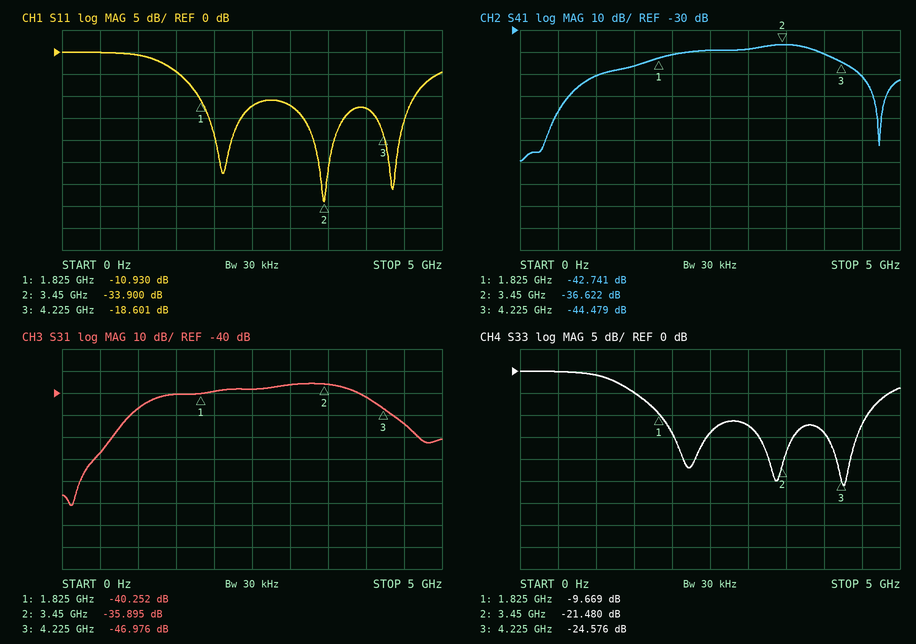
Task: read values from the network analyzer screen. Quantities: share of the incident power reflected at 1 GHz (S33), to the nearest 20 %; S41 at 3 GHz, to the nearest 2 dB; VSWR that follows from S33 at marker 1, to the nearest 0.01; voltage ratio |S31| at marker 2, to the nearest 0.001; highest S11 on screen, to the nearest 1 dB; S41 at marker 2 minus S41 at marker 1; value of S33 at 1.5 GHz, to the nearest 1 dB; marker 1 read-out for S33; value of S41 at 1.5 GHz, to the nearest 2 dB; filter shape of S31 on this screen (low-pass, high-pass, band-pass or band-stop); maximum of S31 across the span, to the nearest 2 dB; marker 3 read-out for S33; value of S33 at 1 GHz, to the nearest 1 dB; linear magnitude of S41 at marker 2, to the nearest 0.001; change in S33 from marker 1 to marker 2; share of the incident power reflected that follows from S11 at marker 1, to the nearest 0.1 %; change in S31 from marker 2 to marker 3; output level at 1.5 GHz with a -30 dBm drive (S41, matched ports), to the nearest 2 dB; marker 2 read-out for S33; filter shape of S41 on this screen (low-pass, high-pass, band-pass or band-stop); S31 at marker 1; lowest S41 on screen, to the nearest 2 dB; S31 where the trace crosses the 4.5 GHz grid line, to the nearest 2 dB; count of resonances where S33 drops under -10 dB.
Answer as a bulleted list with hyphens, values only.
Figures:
- 80 %
- -38 dB
- 1.98
- 0.016
- 0 dB
- 6.119 dB
- -5 dB
- -9.669 dB
- -46 dB
- band-pass
- -36 dB
- -24.576 dB
- -1 dB
- 0.015
- -11.811 dB
- 8.1 %
- -11.081 dB
- -76 dBm
- -21.480 dB
- band-pass
- -40.252 dB
- -90 dB
- -54 dB
- 3
